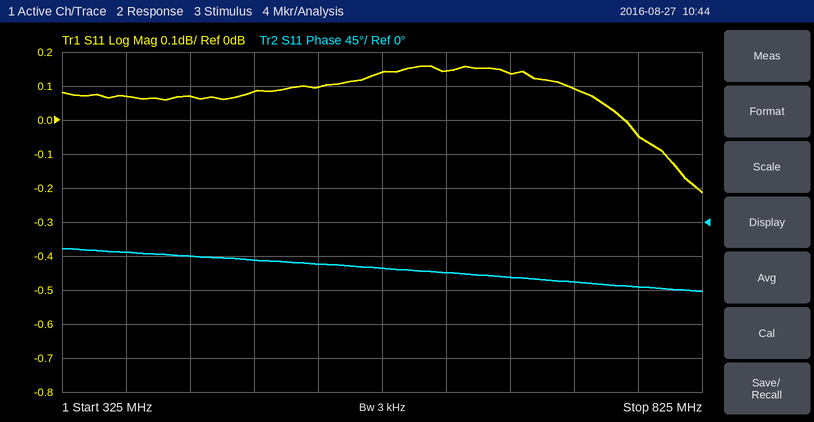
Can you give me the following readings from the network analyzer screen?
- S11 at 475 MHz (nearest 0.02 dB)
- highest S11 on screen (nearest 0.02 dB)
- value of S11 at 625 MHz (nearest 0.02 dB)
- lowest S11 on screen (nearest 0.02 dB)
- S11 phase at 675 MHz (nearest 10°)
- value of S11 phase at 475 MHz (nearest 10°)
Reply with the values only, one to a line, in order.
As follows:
0.08 dB
0.16 dB
0.14 dB
-0.22 dB
-70°
-50°
